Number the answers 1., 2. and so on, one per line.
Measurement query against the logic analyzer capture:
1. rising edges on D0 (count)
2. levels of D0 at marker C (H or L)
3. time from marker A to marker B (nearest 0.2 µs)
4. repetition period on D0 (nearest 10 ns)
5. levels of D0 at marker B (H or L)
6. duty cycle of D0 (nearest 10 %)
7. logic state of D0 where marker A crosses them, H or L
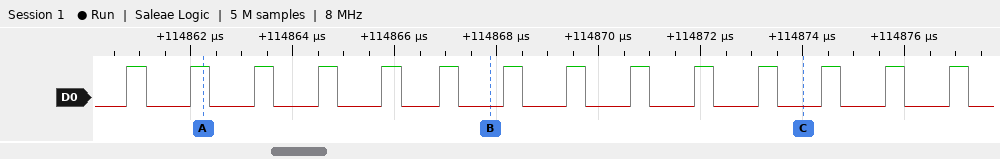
1. 14
2. D0=L
3. 5.6 µs
4. 1240 ns
5. D0=L
6. 30 %
7. D0=H
